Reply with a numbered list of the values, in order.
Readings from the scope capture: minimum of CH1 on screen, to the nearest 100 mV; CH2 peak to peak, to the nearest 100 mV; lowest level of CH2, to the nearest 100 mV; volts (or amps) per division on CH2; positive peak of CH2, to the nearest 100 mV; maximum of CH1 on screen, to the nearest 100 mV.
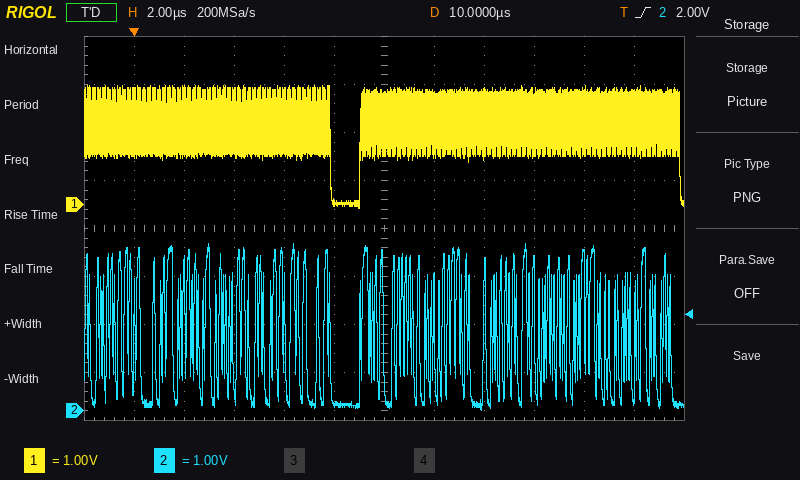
1. -100 mV
2. 3.5 V
3. 0.0 V
4. 1 V
5. 3.5 V
6. 2.5 V
